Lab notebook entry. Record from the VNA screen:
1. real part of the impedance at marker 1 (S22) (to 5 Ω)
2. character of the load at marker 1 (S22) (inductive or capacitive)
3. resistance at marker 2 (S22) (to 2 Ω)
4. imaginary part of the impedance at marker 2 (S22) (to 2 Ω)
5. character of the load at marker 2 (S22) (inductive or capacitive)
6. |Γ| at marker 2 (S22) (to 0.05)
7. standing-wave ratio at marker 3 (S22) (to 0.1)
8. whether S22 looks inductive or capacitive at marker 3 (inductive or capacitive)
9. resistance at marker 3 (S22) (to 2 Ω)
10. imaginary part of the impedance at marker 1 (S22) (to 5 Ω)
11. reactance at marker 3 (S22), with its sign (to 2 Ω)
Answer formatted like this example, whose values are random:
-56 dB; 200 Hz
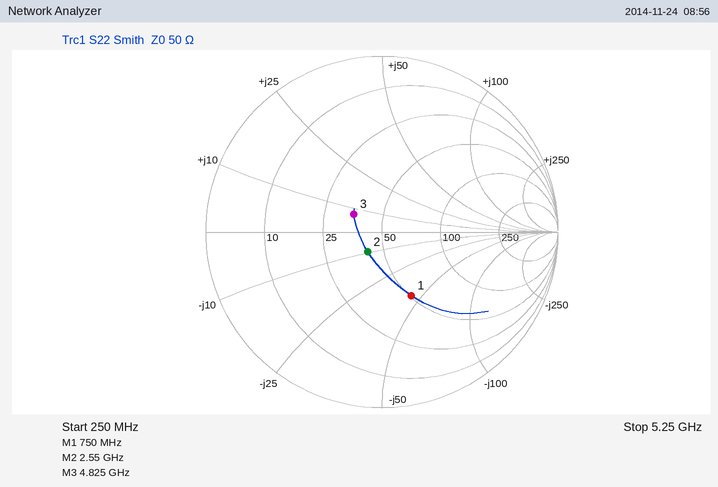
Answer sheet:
50 Ω; capacitive; 42 Ω; -10 Ω; capacitive; 0.15; 1.5; inductive; 36 Ω; -45 Ω; +8 Ω
